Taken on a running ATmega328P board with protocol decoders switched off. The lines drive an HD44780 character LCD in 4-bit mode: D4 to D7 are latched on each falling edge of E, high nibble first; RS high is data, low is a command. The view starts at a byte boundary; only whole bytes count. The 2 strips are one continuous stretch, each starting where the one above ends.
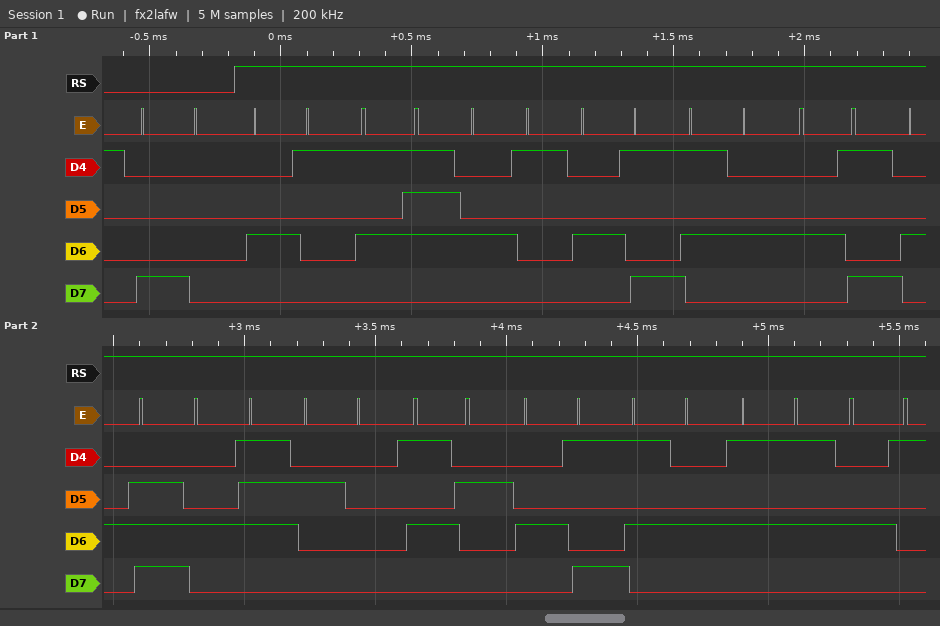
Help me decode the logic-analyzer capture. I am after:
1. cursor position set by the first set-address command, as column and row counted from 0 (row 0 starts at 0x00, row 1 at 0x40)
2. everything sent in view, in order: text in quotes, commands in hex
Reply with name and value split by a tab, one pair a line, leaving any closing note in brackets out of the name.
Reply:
cursor position set by the first set-address command, as column and row counted from 0	column 0, row 0
everything sent in view, in order: text in quotes, commands in hex	0x80 "AWAITING RITUA"
